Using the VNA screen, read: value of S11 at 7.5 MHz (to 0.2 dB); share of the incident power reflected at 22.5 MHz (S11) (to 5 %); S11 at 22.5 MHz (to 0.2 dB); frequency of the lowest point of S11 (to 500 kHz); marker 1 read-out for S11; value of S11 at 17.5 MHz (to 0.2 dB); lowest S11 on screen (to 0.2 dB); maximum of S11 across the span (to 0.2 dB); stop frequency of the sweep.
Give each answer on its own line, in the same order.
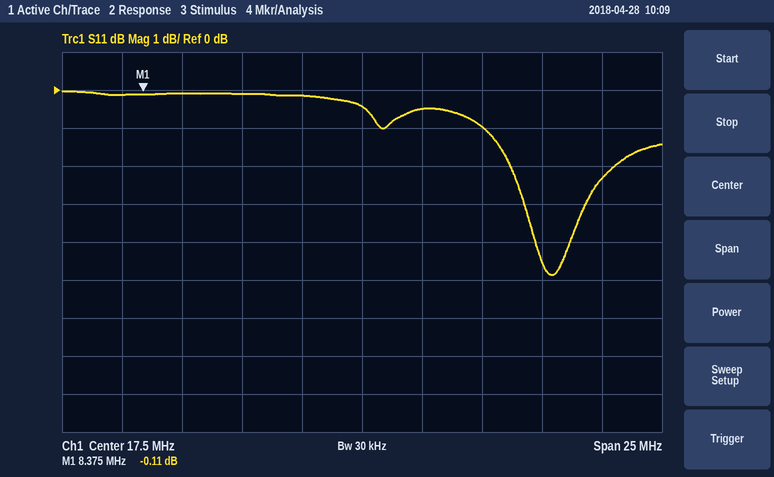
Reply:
-0.2 dB
80 %
-1.0 dB
25.5 MHz
-0.11 dB
-0.4 dB
-4.8 dB
0.0 dB
30 MHz
